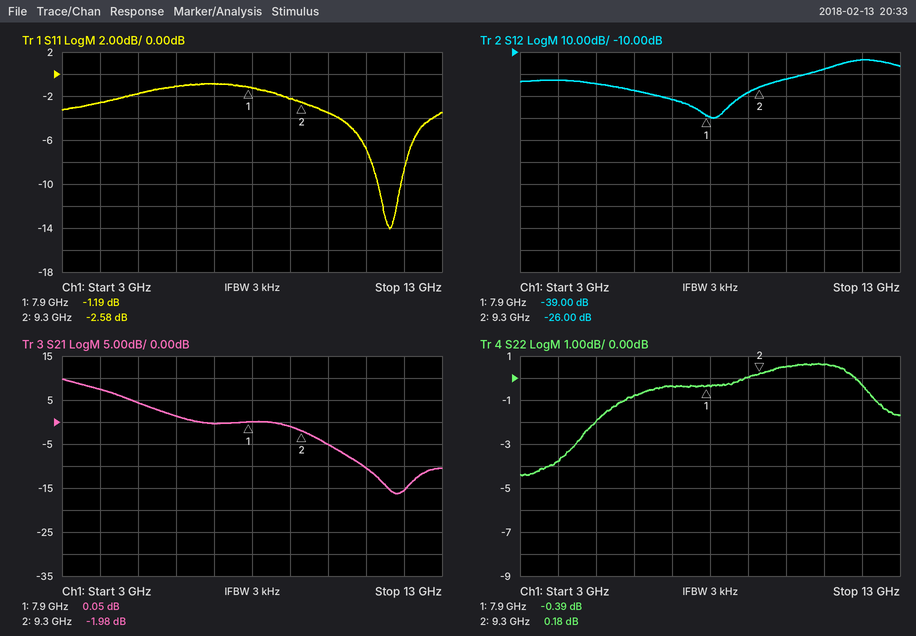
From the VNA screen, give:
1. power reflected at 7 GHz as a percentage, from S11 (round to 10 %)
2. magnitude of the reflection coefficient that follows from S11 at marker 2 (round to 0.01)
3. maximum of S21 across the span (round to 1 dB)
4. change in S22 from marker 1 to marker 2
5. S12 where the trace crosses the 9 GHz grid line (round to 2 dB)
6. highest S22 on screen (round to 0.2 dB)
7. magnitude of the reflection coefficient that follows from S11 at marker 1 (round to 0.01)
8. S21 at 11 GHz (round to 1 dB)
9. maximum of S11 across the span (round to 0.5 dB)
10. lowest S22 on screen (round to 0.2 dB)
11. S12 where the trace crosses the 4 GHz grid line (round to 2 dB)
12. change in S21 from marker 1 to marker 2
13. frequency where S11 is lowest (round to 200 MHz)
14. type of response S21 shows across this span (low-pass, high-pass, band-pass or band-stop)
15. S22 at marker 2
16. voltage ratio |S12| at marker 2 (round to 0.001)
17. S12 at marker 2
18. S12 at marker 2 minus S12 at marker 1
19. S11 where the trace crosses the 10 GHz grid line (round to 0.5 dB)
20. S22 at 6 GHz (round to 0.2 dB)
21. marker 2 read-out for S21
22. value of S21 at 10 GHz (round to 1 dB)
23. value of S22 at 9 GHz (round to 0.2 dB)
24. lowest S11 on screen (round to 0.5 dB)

80 %
0.74
10 dB
0.57 dB
-28 dB
0.6 dB
0.87
-10 dB
-1.0 dB
-4.4 dB
-22 dB
-2.03 dB
11.6 GHz
low-pass
0.18 dB
0.050
-26.00 dB
13.00 dB
-3.5 dB
-0.8 dB
-1.98 dB
-5 dB
0.0 dB
-14.0 dB
